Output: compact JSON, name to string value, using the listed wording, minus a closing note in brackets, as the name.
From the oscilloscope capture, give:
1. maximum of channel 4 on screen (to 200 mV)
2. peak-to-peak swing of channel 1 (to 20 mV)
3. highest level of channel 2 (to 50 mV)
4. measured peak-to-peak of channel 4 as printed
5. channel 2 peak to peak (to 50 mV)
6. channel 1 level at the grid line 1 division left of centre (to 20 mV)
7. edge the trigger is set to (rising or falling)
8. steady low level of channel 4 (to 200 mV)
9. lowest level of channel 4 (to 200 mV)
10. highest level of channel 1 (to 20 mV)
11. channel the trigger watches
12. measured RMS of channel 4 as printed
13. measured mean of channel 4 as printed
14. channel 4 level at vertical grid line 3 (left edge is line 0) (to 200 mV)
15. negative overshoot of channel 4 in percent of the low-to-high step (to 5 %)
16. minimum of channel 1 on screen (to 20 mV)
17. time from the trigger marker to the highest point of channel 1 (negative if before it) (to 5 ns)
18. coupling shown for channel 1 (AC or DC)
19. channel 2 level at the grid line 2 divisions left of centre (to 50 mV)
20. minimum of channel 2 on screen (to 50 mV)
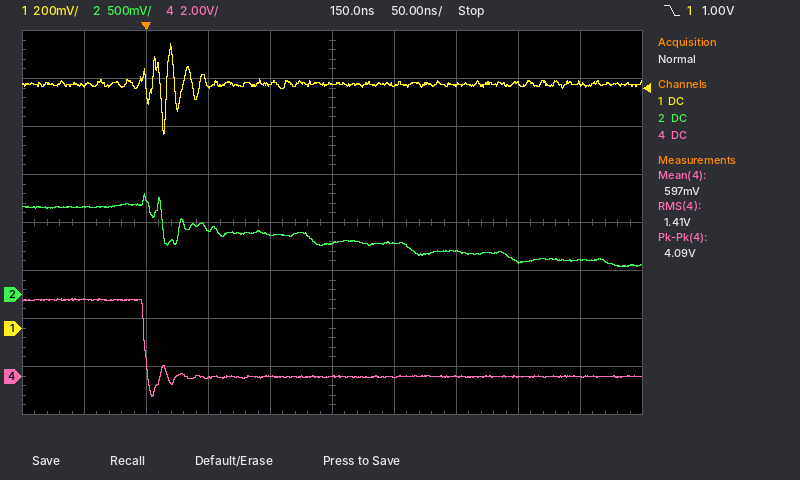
{"maximum of channel 4 on screen": "3.2 V", "peak-to-peak swing of channel 1": "380 mV", "highest level of channel 2": "1.05 V", "measured peak-to-peak of channel 4 as printed": "4.09 V", "channel 2 peak to peak": "750 mV", "channel 1 level at the grid line 1 division left of centre": "1.02 V", "edge the trigger is set to": "falling", "steady low level of channel 4": "0.0 V", "lowest level of channel 4": "-800 mV", "highest level of channel 1": "1.18 V", "channel the trigger watches": "channel 1", "measured RMS of channel 4 as printed": "1.41 V", "measured mean of channel 4 as printed": "597 mV", "channel 4 level at vertical grid line 3 (left edge is line 0)": "0.0 V", "negative overshoot of channel 4 in percent of the low-to-high step": "25 %", "minimum of channel 1 on screen": "800 mV", "time from the trigger marker to the highest point of channel 1 (negative if before it)": "+20 ns", "coupling shown for channel 1": "DC", "channel 2 level at the grid line 2 divisions left of centre": "700 mV", "minimum of channel 2 on screen": "300 mV"}
